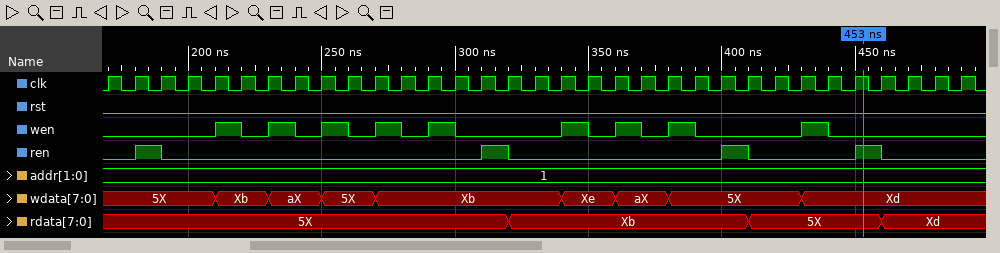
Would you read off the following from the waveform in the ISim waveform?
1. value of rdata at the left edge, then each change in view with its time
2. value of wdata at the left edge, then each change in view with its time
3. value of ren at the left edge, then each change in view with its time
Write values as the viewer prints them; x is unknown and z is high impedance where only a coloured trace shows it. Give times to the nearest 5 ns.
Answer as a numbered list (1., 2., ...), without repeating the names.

1. 5X, Xb at 320 ns, 5X at 410 ns, Xd at 460 ns
2. 5X, Xb at 210 ns, aX at 230 ns, 5X at 250 ns, Xb at 270 ns, Xe at 340 ns, aX at 360 ns, 5X at 380 ns, Xd at 430 ns
3. 0, 1 at 180 ns, 0 at 190 ns, 1 at 310 ns, 0 at 320 ns, 1 at 400 ns, 0 at 410 ns, 1 at 450 ns, 0 at 460 ns
